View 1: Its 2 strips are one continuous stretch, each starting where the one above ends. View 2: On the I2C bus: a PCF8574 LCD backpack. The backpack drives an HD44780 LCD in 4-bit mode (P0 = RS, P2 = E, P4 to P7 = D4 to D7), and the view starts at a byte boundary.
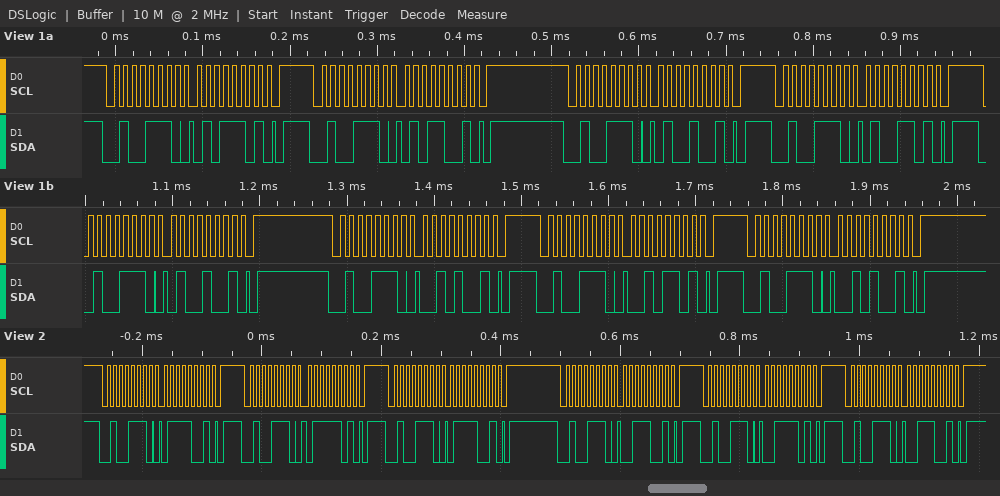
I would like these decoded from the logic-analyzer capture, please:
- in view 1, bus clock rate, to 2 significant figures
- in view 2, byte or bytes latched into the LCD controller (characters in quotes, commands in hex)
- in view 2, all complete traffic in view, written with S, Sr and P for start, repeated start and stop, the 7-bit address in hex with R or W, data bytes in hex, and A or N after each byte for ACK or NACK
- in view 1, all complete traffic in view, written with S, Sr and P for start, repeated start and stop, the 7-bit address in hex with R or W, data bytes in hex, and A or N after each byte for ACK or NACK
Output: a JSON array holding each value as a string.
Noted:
["100 kHz", "'s'", "S 27W A 79 A P S 27W A 7D A P S 27W A 79 A P S 27W A 39 A P S 27W A 3D A P S 27W A 39 A P", "S 27W A 5D A P S 27W A 59 A P S 27W A 49 A P S 27W A 4D A P S 27W A 49 A P S 27W A 29 A P S 27W A 2D A P S 27W A 29 A P"]
